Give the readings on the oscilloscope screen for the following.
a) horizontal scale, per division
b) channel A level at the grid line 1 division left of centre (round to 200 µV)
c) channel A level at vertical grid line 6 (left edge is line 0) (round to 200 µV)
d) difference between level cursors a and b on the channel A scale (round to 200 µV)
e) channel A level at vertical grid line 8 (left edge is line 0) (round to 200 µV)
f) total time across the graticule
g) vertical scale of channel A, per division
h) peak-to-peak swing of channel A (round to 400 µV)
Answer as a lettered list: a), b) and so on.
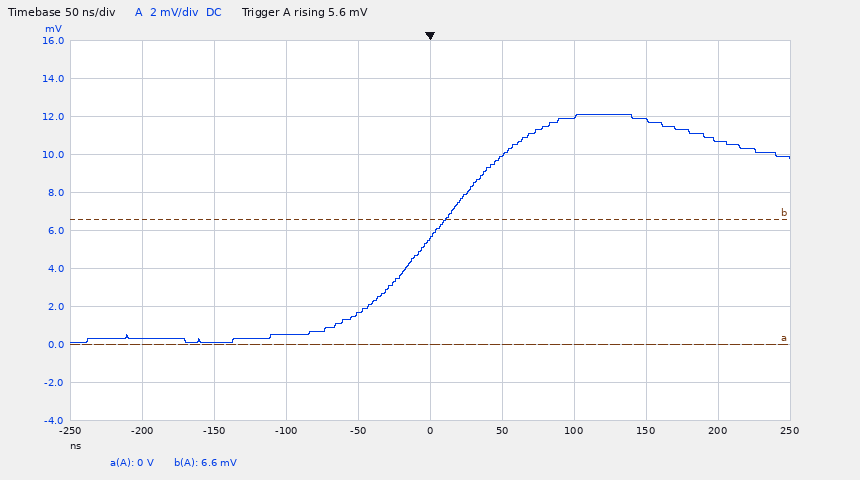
a) 50 ns
b) 1.6 mV
c) 10.0 mV
d) 6.6 mV
e) 11.8 mV
f) 500 ns
g) 2 mV
h) 12.0 mV
